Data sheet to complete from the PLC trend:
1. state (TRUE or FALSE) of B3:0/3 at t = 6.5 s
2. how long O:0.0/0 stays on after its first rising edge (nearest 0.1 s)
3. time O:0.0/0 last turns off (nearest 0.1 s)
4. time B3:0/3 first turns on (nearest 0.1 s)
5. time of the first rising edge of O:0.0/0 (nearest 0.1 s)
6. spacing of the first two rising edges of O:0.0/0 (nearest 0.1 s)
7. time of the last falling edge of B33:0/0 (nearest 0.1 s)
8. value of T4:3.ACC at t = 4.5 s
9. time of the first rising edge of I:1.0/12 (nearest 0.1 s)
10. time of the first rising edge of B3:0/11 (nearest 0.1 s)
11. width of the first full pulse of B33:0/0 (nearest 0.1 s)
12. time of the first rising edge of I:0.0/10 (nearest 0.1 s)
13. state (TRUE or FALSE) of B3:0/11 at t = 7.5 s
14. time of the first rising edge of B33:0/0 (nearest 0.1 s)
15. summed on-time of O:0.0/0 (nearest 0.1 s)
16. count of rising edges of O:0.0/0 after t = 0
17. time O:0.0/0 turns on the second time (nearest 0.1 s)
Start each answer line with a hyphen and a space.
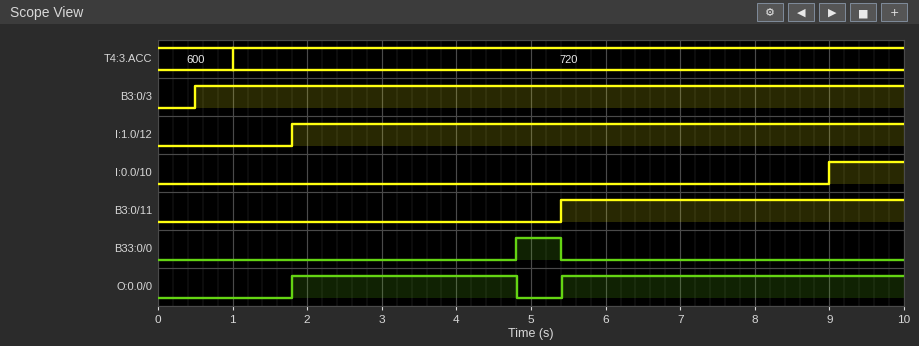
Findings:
- TRUE
- 3.0 s
- 4.8 s
- 0.5 s
- 1.8 s
- 3.6 s
- 5.4 s
- 720
- 1.8 s
- 5.4 s
- 0.6 s
- 9.0 s
- TRUE
- 4.8 s
- 7.6 s
- 2
- 5.4 s
